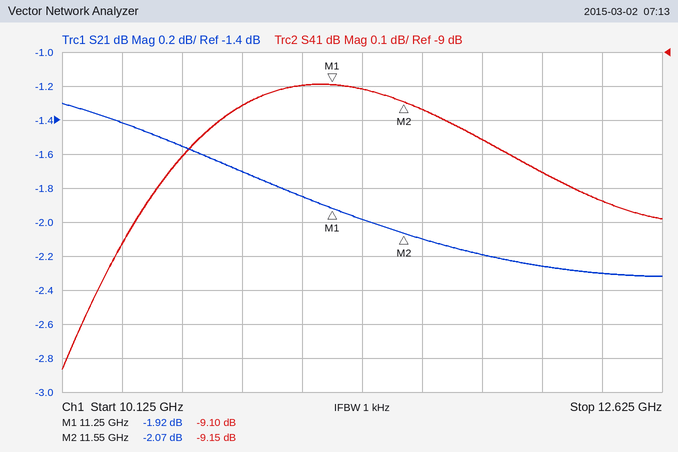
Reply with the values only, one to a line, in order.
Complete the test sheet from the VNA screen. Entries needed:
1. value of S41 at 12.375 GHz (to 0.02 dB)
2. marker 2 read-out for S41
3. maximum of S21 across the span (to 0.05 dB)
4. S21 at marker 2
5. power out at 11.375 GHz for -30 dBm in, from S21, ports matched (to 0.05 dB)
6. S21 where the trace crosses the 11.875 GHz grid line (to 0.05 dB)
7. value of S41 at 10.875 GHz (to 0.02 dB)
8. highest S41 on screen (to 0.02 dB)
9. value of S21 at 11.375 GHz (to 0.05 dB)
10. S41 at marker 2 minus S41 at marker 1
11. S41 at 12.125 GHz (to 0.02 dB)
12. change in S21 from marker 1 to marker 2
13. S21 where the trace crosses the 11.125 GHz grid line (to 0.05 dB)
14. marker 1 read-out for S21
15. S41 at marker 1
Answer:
-9.44 dB
-9.15 dB
-1.30 dB
-2.07 dB
-32.00 dBm
-2.20 dB
-9.16 dB
-9.10 dB
-2.00 dB
-0.05 dB
-9.36 dB
-0.15 dB
-1.85 dB
-1.92 dB
-9.10 dB
